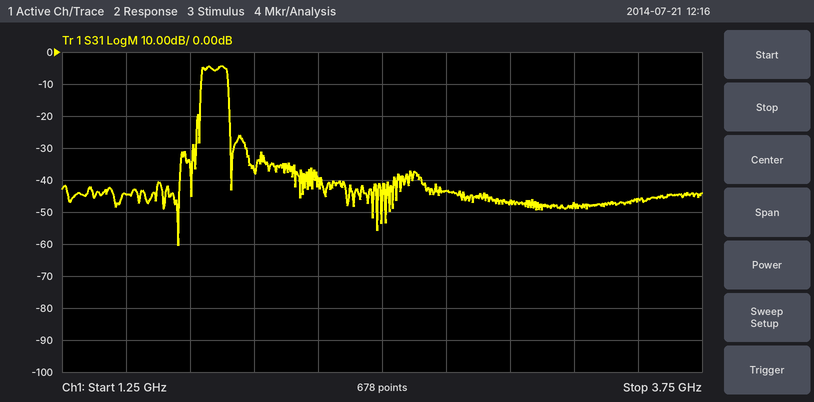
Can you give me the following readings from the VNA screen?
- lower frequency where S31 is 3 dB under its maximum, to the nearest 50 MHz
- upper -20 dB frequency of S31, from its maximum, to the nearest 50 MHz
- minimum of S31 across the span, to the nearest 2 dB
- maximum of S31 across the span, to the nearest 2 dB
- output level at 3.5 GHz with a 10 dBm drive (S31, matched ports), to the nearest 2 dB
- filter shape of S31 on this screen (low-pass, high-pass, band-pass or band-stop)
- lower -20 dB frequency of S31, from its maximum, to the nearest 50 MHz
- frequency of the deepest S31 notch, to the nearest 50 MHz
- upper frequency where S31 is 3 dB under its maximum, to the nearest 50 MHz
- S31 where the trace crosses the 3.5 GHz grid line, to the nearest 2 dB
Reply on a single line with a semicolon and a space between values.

1.80 GHz; 1.90 GHz; -60 dB; -4 dB; -36 dBm; band-pass; 1.80 GHz; 1.70 GHz; 1.90 GHz; -46 dB
